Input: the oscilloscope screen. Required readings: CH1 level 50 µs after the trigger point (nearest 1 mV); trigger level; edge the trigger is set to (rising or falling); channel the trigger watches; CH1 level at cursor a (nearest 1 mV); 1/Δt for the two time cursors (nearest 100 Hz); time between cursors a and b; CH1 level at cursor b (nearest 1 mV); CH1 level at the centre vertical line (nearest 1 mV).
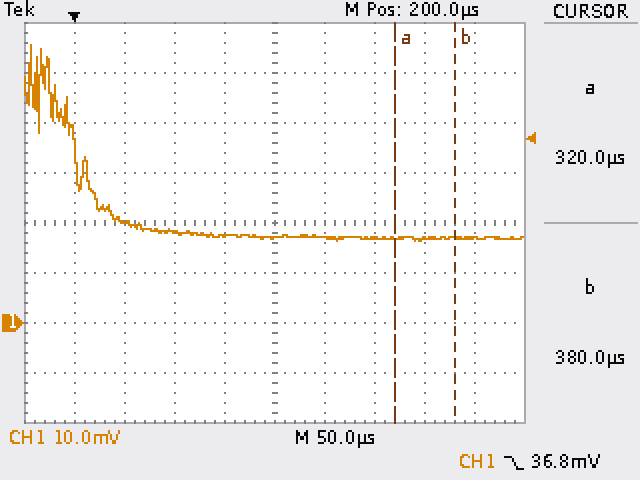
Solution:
20 mV
36.8 mV
falling
CH1
17 mV
16.7 kHz
60 µs
17 mV
17 mV
